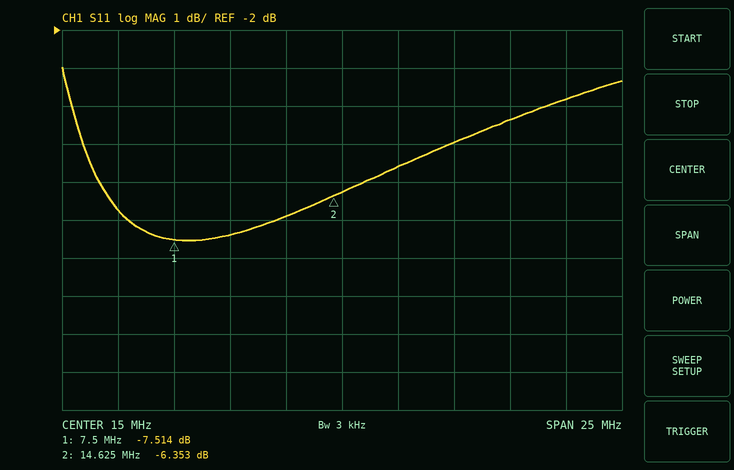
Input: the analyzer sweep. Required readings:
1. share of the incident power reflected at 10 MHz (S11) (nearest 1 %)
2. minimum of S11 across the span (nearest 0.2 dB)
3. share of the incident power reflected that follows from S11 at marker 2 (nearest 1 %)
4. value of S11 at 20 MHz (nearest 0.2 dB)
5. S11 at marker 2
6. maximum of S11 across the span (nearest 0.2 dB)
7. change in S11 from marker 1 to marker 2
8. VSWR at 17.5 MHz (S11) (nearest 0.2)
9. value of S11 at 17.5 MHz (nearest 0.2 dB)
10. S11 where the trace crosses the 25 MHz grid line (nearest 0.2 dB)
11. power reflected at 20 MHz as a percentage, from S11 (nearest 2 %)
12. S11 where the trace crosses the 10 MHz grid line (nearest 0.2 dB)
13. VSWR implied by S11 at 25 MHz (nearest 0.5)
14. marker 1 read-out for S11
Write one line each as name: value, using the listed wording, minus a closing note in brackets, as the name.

share of the incident power reflected at 10 MHz (S11): 18 %
minimum of S11 across the span: -7.6 dB
share of the incident power reflected that follows from S11 at marker 2: 23 %
value of S11 at 20 MHz: -5.0 dB
S11 at marker 2: -6.353 dB
maximum of S11 across the span: -3.0 dB
change in S11 from marker 1 to marker 2: 1.161 dB
VSWR at 17.5 MHz (S11): 3.2
value of S11 at 17.5 MHz: -5.6 dB
S11 where the trace crosses the 25 MHz grid line: -3.8 dB
power reflected at 20 MHz as a percentage, from S11: 32 %
S11 where the trace crosses the 10 MHz grid line: -7.4 dB
VSWR implied by S11 at 25 MHz: 4.5
marker 1 read-out for S11: -7.514 dB
